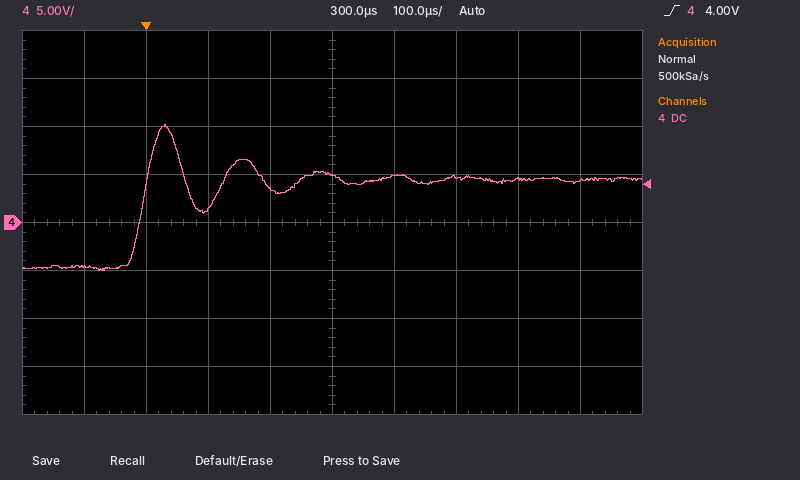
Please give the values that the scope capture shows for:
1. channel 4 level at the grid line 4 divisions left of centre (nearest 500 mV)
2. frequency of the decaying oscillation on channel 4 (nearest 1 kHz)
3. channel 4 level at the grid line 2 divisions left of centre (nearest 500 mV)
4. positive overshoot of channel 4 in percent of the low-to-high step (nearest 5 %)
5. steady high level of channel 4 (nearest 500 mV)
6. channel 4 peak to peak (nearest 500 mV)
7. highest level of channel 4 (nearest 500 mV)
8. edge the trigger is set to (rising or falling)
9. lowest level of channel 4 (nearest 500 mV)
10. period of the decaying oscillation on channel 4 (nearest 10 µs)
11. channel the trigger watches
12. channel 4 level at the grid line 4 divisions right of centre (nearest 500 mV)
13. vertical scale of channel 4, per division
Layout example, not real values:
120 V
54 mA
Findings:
-4.5 V
8 kHz
1.5 V
60 %
4.5 V
15.0 V
10.0 V
rising
-5.0 V
130 µs
channel 4
4.5 V
5 V
